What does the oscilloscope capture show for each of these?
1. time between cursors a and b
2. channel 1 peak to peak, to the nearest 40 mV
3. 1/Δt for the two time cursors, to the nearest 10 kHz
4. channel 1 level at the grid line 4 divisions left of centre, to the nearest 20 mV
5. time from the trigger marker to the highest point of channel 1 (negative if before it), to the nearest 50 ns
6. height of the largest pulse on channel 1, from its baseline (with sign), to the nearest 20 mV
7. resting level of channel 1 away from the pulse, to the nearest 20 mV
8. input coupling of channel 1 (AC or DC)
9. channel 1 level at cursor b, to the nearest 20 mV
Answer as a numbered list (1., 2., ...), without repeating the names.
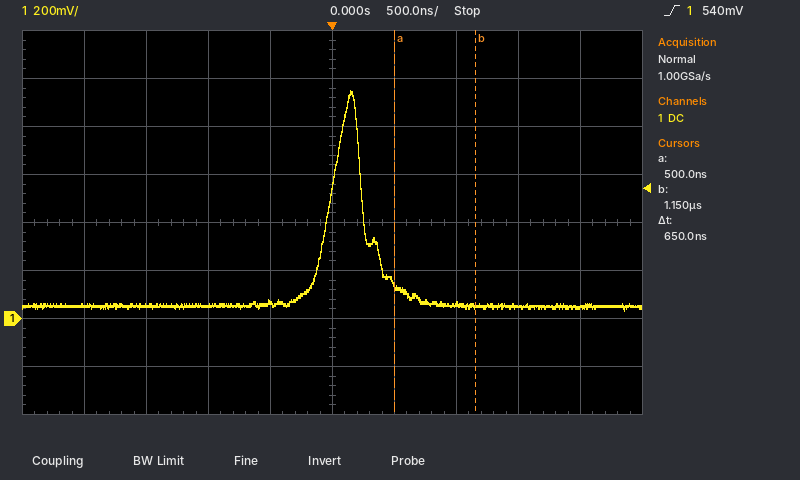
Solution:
1. 650 ns
2. 920 mV
3. 1.54 MHz
4. 60 mV
5. +150 ns
6. +900 mV
7. 60 mV
8. DC
9. 60 mV
